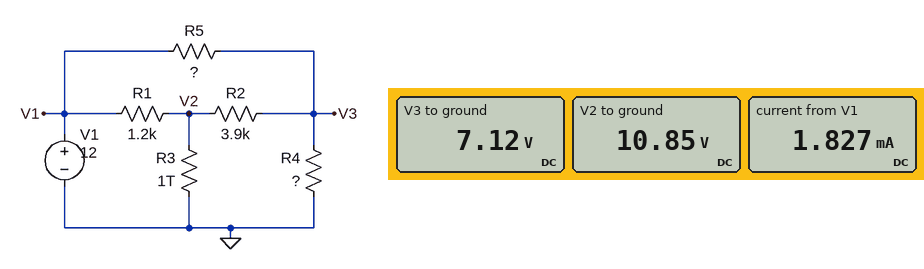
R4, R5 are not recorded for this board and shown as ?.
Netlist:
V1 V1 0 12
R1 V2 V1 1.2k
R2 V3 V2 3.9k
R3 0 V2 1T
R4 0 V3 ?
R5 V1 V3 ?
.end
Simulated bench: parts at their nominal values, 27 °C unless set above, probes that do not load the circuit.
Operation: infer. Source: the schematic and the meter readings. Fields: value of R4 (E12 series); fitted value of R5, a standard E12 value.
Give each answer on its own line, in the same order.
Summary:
3.9 kΩ
5.6 kΩ
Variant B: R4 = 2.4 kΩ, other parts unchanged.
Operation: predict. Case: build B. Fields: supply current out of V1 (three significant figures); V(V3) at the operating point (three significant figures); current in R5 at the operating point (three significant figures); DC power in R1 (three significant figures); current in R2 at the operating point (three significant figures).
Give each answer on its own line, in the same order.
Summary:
2.37 mA
5.68 V
1.13 mA
1.84 mW
1.24 mA
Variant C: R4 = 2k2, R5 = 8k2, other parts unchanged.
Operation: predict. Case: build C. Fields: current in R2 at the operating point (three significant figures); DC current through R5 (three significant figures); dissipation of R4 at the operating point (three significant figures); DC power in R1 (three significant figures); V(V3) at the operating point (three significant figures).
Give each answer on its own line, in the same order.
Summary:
1.38 mA
861 µA
11.1 mW
2.30 mW
4.94 V
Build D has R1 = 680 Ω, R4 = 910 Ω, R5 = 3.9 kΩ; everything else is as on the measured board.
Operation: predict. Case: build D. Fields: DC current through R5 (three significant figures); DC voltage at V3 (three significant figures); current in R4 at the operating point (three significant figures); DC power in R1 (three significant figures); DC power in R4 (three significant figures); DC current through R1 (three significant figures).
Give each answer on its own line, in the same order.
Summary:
2.15 mA
3.62 V
3.98 mA
2.28 mW
14.4 mW
1.83 mA
